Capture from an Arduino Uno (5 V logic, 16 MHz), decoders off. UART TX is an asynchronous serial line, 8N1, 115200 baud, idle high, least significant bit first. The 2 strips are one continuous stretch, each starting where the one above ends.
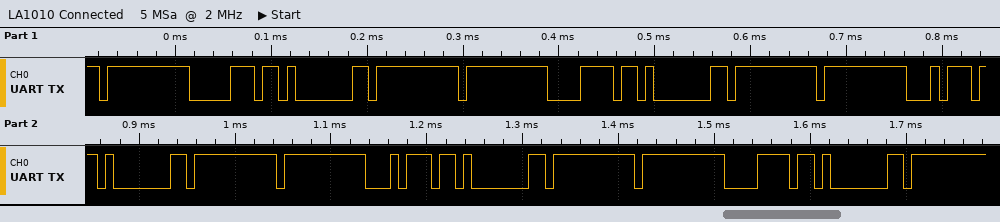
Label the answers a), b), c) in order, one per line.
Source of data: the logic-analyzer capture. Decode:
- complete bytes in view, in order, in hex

a) 0xFF 0x70 0x01 0xFF 0xFF 0x78 0x01 0xFF 0xFF 0x74 0x01 0xFF 0xFF 0x74 0x01 0xFF 0xFF 0x78 0x01 0xFF
